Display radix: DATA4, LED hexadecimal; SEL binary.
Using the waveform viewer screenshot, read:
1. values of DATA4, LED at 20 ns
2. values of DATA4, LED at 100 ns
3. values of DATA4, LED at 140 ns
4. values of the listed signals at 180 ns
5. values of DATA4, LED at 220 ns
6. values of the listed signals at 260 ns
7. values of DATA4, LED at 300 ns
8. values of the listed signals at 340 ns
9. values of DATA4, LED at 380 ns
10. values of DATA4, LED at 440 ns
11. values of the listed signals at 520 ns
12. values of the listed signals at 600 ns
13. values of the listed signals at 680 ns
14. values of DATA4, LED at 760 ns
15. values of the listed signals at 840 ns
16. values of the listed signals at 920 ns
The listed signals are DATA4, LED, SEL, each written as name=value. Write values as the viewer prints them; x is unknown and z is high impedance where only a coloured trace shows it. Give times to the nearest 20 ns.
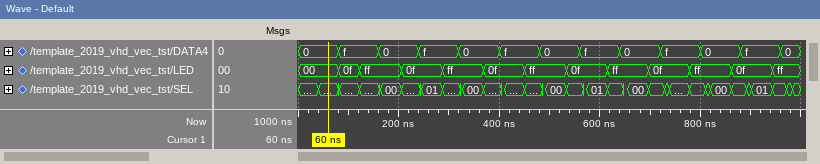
DATA4=0, LED=00
DATA4=f, LED=0f
DATA4=f, LED=ff
DATA4=0, LED=ff, SEL=00
DATA4=0, LED=0f
DATA4=f, LED=0f, SEL=01
DATA4=f, LED=ff
DATA4=0, LED=ff, SEL=00
DATA4=0, LED=0f
DATA4=f, LED=0f
DATA4=0, LED=ff, SEL=00
DATA4=f, LED=0f, SEL=01
DATA4=0, LED=ff, SEL=00
DATA4=f, LED=0f
DATA4=0, LED=ff, SEL=00
DATA4=f, LED=0f, SEL=01
